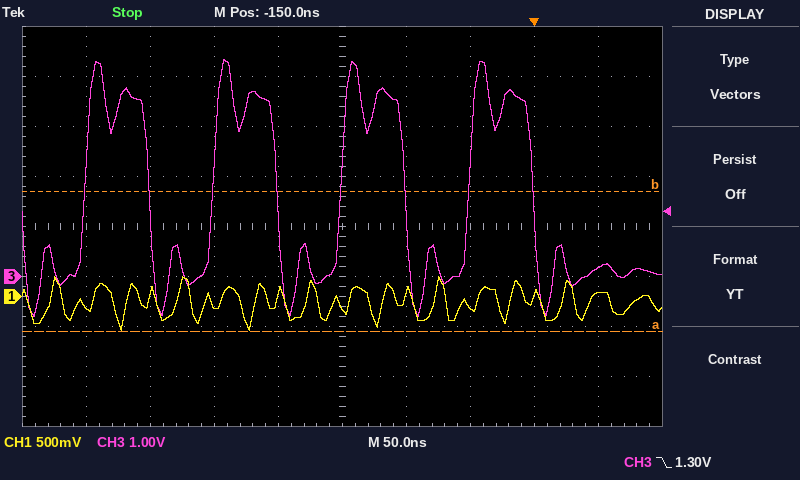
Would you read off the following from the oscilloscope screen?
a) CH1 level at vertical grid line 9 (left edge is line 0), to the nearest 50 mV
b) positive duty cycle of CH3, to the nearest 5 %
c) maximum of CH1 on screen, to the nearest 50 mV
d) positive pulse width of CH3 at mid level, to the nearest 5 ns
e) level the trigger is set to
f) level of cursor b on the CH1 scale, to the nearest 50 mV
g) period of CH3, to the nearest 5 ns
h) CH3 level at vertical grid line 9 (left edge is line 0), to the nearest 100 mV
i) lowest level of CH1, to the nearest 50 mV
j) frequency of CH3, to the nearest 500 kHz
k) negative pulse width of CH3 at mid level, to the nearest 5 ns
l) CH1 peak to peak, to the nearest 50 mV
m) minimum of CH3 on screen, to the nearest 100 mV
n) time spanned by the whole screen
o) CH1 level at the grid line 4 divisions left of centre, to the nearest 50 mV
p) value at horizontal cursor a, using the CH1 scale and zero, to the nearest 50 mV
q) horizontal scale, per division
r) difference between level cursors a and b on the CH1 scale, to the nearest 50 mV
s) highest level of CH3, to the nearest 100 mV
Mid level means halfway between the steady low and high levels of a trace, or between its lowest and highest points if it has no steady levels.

50 mV
50 %
200 mV
50 ns
1.30 V
1.05 V
100 ns
200 mV
-350 mV
10.0 MHz
50 ns
550 mV
-800 mV
500 ns
-100 mV
-350 mV
50 ns
1.40 V
4.3 V
